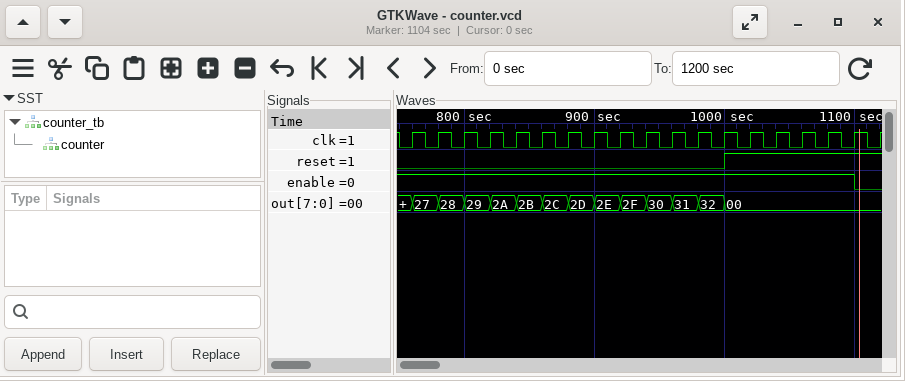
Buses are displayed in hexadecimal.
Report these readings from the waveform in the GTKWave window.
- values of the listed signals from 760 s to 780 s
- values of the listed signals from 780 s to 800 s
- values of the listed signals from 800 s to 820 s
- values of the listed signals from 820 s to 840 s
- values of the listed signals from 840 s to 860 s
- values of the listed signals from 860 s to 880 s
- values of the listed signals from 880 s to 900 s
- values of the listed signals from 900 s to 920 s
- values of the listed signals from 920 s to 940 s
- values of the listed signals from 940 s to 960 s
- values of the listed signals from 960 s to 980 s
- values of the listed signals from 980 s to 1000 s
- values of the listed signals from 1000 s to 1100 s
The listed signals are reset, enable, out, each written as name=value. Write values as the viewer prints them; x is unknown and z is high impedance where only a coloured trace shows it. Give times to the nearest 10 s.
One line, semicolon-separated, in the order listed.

reset=0, enable=1, out=27; reset=0, enable=1, out=28; reset=0, enable=1, out=29; reset=0, enable=1, out=2A; reset=0, enable=1, out=2B; reset=0, enable=1, out=2C; reset=0, enable=1, out=2D; reset=0, enable=1, out=2E; reset=0, enable=1, out=2F; reset=0, enable=1, out=30; reset=0, enable=1, out=31; reset=0, enable=1, out=32; reset=1, enable=1, out=00
